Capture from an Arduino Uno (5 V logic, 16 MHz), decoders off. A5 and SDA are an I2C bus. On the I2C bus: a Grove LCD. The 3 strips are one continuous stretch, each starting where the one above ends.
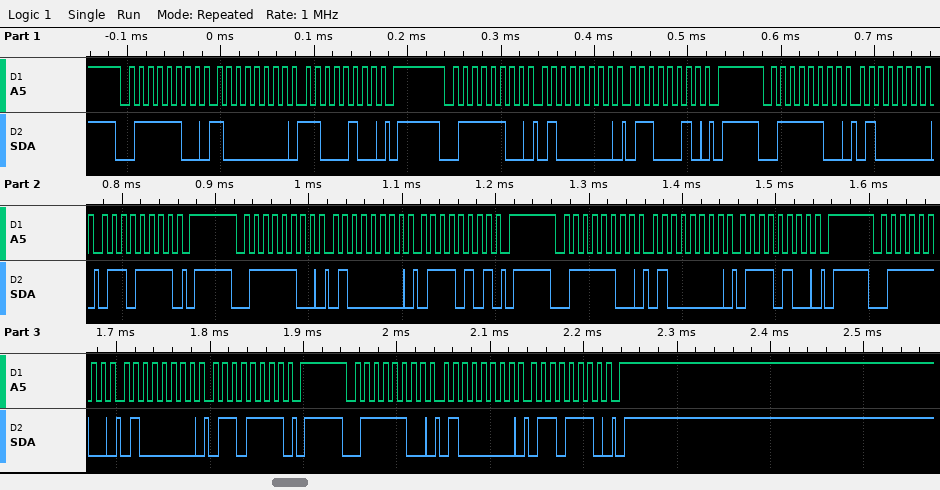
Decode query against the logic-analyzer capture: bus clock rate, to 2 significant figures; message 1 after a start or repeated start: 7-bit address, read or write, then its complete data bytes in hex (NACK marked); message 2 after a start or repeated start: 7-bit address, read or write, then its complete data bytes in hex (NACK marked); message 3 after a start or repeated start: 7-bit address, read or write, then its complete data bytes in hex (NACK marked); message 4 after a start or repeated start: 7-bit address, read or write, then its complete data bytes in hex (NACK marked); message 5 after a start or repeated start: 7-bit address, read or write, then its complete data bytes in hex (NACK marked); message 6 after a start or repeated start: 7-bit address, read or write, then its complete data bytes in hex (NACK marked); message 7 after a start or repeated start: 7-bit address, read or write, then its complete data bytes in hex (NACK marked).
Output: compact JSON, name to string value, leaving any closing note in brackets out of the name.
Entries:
{"bus clock rate, to 2 significant figures": "100 kHz", "message 1 after a start or repeated start: 7-bit address, read or write, then its complete data bytes in hex": "0x3E write: 80 C4", "message 2 after a start or repeated start: 7-bit address, read or write, then its complete data bytes in hex": "0x3E write: 40 62", "message 3 after a start or repeated start: 7-bit address, read or write, then its complete data bytes in hex": "0x3E write: 40 6F", "message 4 after a start or repeated start: 7-bit address, read or write, then its complete data bytes in hex": "0x3E write: 40 75", "message 5 after a start or repeated start: 7-bit address, read or write, then its complete data bytes in hex": "0x3E write: 40 74", "message 6 after a start or repeated start: 7-bit address, read or write, then its complete data bytes in hex": "0x3E write: 40 6F", "message 7 after a start or repeated start: 7-bit address, read or write, then its complete data bytes in hex": "0x3E write: 40 6E"}
